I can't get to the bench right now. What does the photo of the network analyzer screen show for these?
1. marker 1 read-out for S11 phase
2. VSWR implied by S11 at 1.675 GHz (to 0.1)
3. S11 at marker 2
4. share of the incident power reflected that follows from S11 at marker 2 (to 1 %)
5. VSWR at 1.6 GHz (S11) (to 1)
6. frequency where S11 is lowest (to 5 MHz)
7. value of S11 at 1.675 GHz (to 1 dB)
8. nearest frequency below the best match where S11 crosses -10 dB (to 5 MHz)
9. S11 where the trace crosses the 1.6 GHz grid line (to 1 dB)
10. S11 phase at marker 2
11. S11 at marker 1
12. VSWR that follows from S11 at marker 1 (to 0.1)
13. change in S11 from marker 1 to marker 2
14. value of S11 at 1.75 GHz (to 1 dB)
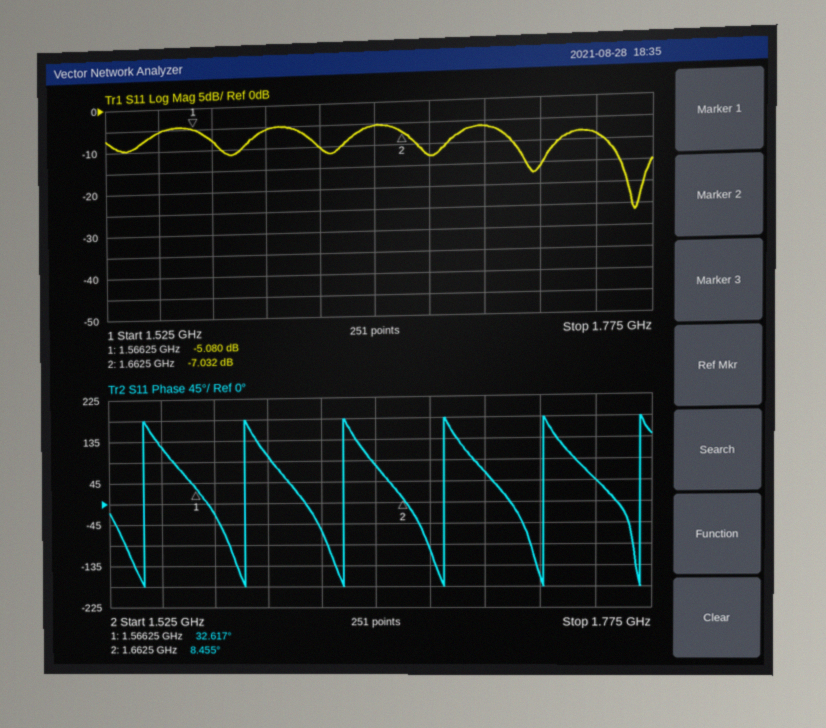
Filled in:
32.617°
1.6
-7.032 dB
20 %
3
1.765 GHz
-13 dB
1.755 GHz
-6 dB
8.455°
-5.080 dB
3.5
-1.952 dB
-9 dB
